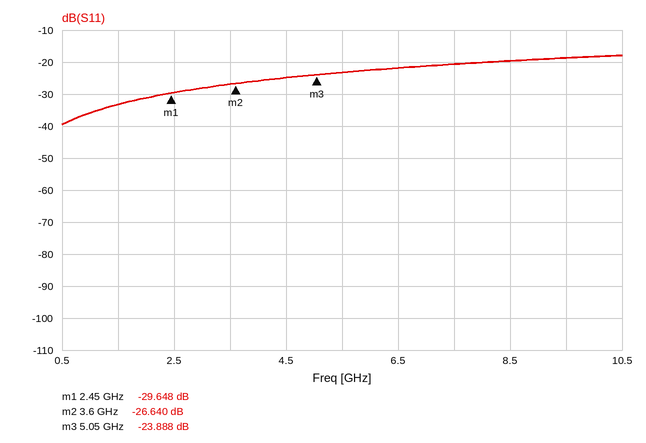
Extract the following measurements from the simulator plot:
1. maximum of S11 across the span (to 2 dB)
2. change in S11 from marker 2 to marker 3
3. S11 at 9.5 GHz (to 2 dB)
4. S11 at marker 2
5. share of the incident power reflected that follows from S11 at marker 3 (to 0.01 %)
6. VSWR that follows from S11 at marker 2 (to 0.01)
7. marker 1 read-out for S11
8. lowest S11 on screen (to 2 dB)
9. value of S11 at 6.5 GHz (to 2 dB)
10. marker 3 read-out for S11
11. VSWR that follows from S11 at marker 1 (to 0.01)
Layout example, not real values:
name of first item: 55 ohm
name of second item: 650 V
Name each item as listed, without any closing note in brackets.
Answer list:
maximum of S11 across the span: -18 dB
change in S11 from marker 2 to marker 3: 2.752 dB
S11 at 9.5 GHz: -18 dB
S11 at marker 2: -26.640 dB
share of the incident power reflected that follows from S11 at marker 3: 0.41 %
VSWR that follows from S11 at marker 2: 1.10
marker 1 read-out for S11: -29.648 dB
lowest S11 on screen: -40 dB
value of S11 at 6.5 GHz: -22 dB
marker 3 read-out for S11: -23.888 dB
VSWR that follows from S11 at marker 1: 1.07
